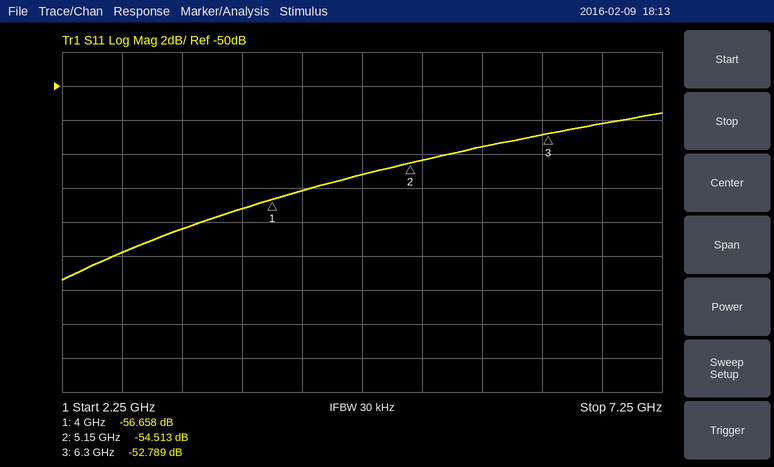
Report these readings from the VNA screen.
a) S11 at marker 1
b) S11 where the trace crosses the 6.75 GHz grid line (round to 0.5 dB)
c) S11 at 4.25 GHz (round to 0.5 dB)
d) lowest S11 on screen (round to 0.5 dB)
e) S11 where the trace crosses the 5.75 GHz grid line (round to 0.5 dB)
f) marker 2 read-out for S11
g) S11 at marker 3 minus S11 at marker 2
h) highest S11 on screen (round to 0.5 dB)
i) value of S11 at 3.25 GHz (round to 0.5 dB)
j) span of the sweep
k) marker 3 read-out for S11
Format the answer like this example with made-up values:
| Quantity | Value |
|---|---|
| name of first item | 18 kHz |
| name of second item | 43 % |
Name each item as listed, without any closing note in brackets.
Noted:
| Quantity | Value |
|---|---|
| S11 at marker 1 | -56.658 dB |
| S11 where the trace crosses the 6.75 GHz grid line | -52.0 dB |
| S11 at 4.25 GHz | -56.0 dB |
| lowest S11 on screen | -61.5 dB |
| S11 where the trace crosses the 5.75 GHz grid line | -53.5 dB |
| marker 2 read-out for S11 | -54.513 dB |
| S11 at marker 3 minus S11 at marker 2 | 1.724 dB |
| highest S11 on screen | -51.5 dB |
| value of S11 at 3.25 GHz | -58.5 dB |
| span of the sweep | 5 GHz |
| marker 3 read-out for S11 | -52.789 dB |
